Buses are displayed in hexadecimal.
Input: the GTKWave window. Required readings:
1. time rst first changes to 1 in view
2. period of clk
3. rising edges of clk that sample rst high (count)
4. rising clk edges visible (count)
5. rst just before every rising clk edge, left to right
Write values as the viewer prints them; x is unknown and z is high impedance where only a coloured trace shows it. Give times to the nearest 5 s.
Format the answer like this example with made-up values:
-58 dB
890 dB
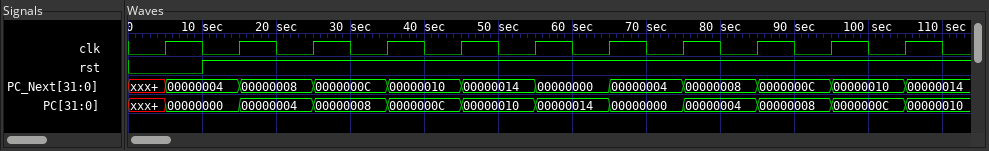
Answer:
10 s
10 s
10
11
0 1 1 1 1 1 1 1 1 1 1
